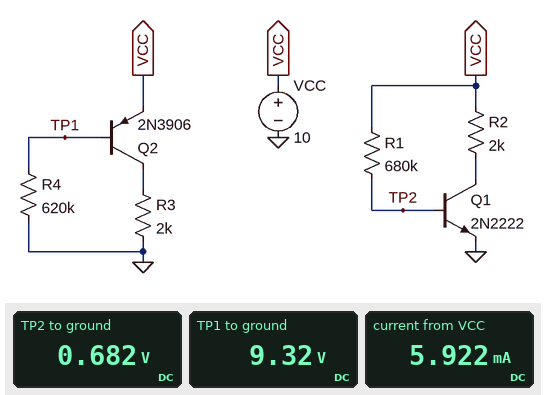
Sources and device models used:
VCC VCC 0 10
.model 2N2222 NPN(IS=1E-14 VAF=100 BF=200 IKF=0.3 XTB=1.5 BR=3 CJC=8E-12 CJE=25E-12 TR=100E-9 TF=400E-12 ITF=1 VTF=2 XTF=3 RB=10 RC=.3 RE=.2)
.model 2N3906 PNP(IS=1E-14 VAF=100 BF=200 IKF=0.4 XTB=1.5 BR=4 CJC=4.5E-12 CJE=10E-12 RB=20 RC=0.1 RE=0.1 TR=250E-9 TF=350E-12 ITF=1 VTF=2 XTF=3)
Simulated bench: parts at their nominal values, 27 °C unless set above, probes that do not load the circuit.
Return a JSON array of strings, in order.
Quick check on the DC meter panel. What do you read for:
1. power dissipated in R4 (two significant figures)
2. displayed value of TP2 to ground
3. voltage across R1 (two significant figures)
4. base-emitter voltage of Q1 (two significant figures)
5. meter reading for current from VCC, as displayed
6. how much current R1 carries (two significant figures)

["140 µW", "0.682 V", "9.3 V", "680 mV", "5.922 mA", "14 µA"]
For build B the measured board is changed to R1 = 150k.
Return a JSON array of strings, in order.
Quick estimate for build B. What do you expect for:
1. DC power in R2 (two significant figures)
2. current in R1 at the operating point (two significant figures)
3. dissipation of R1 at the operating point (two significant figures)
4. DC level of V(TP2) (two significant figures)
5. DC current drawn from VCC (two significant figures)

["49 mW", "62 µA", "580 µW", "700 mV", "8.1 mA"]
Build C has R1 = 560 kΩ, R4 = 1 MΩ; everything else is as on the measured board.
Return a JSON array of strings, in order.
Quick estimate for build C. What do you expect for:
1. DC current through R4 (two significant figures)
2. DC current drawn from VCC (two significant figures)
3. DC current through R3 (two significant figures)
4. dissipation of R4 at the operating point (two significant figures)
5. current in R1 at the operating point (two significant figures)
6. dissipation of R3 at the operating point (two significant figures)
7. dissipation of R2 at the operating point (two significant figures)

["9.3 µA", "5.4 mA", "2.0 mA", "87 µW", "17 µA", "7.7 mW", "23 mW"]
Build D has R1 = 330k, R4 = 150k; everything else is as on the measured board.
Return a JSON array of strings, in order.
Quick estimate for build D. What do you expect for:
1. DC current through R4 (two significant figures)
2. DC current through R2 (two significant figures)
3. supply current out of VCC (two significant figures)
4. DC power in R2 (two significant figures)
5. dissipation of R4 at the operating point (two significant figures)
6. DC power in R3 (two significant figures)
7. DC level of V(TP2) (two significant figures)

["62 µA", "4.9 mA", "10 mA", "48 mW", "580 µW", "49 mW", "700 mV"]
